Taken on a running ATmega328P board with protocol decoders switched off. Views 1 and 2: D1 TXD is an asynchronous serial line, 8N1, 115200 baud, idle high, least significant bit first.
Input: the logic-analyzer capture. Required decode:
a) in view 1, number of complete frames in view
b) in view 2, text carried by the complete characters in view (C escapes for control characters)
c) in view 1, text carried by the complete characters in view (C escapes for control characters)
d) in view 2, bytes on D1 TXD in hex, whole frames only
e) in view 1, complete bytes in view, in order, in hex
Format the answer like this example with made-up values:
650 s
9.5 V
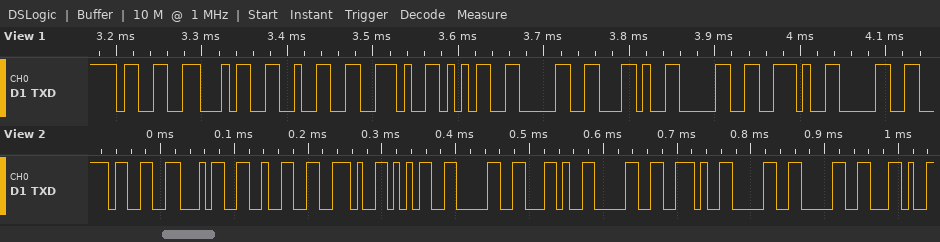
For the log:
10
"342.50,0.00,"
"342.50,0.0"
33 34 32 2E 35 30 2C 30 2E 30 30 2C
33 34 32 2E 35 30 2C 30 2E 30
